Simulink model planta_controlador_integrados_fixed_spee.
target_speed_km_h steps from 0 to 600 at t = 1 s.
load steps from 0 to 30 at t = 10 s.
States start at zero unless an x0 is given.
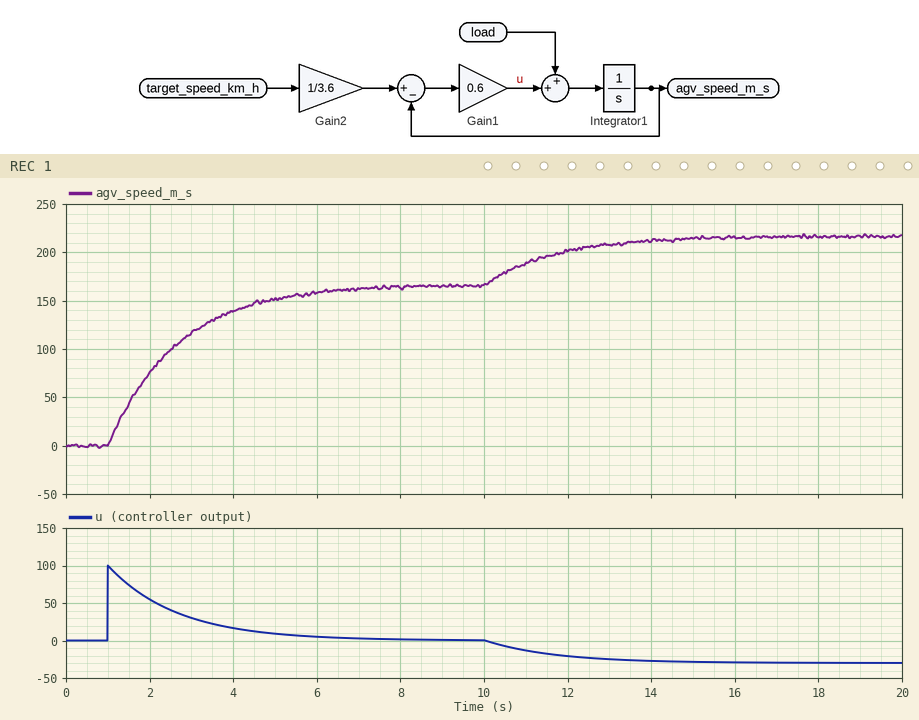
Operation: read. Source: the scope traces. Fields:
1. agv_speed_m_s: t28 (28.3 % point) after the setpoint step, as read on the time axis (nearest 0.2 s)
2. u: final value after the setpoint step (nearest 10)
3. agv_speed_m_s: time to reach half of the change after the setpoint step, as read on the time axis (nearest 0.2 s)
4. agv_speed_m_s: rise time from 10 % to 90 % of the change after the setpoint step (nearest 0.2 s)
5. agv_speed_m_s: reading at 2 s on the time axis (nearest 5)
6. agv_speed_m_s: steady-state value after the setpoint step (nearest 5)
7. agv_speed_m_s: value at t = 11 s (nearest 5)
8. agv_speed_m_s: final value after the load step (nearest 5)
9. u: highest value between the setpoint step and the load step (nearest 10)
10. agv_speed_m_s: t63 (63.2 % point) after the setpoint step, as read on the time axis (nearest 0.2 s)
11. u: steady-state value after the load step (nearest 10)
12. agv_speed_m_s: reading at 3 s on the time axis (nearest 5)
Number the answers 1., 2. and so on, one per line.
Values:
1. 1.6 s
2. 0
3. 2.2 s
4. 3.6 s
5. 75
6. 165
7. 190
8. 215
9. 100
10. 2.6 s
11. -30
12. 115
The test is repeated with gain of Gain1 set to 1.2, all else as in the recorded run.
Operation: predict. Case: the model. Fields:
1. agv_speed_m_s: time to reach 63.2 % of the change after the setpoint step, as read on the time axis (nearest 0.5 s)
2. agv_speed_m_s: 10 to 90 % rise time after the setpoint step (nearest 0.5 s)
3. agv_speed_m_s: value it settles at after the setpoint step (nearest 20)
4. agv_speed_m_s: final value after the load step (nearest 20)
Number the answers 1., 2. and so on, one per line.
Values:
1. 2.0 s
2. 2.0 s
3. 160
4. 200
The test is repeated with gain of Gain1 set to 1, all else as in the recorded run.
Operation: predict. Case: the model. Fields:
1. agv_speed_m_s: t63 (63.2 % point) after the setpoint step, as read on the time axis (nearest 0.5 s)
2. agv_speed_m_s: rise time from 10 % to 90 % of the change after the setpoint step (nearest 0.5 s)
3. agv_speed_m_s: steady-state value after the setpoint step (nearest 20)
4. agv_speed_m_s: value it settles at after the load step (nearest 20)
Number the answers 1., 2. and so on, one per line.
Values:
1. 2.0 s
2. 2.0 s
3. 160
4. 200
